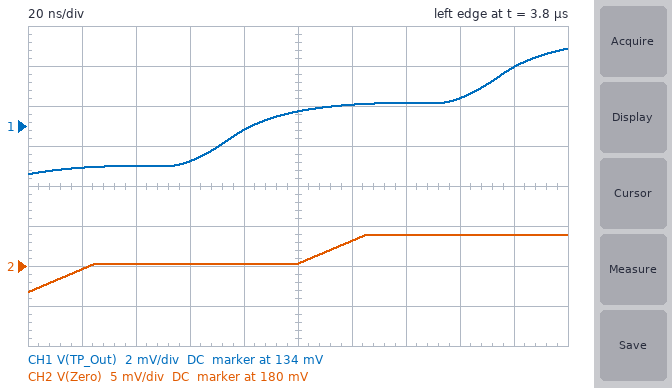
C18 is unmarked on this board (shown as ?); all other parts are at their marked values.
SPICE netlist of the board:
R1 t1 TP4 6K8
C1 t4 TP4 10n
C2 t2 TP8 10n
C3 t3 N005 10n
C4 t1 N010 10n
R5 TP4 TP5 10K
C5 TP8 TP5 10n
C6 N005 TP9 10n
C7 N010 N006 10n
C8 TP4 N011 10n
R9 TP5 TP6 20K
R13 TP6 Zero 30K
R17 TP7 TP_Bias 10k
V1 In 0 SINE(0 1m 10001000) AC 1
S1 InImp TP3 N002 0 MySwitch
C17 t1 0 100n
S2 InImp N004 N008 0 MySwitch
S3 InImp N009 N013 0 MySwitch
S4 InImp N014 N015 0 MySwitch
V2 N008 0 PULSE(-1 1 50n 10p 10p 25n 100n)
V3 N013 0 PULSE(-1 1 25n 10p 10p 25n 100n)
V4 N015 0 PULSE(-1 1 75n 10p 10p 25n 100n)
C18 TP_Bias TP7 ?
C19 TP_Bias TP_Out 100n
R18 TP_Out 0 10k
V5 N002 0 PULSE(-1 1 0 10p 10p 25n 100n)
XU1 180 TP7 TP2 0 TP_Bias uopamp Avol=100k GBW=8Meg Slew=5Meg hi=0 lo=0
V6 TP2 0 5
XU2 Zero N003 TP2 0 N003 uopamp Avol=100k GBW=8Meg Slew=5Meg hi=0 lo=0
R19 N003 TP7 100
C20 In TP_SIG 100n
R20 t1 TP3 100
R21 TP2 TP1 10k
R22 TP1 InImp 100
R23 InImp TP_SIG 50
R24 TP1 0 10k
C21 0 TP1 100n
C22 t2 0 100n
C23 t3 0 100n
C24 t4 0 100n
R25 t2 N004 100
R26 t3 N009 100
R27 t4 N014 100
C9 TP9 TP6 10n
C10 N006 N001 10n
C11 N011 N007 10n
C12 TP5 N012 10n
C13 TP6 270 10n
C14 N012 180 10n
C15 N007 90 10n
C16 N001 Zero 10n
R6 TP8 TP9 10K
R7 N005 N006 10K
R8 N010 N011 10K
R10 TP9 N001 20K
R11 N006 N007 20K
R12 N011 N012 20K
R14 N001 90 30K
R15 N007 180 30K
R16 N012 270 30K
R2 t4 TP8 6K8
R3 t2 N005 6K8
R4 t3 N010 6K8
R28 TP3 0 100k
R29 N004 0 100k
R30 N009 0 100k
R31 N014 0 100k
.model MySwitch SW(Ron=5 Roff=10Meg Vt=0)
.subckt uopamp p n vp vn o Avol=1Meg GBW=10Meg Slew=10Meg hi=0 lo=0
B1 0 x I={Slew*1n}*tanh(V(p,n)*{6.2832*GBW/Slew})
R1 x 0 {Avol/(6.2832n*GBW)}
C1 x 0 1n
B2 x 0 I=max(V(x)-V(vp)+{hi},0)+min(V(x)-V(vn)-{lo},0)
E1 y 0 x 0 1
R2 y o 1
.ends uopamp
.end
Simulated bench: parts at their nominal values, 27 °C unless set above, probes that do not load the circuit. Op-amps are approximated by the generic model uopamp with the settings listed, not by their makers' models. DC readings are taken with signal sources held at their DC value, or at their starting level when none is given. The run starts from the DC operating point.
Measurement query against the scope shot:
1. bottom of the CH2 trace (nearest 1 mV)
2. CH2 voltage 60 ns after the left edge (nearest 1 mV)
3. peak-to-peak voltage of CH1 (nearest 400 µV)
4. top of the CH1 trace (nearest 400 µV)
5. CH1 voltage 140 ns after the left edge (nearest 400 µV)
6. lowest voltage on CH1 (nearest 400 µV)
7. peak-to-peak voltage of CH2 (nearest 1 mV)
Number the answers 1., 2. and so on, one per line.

1. 177 mV
2. 180 mV
3. 6.4 mV
4. 138.0 mV
5. 135.2 mV
6. 131.6 mV
7. 7 mV
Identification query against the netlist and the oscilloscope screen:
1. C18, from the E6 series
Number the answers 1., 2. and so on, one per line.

1. 3.3 nF
